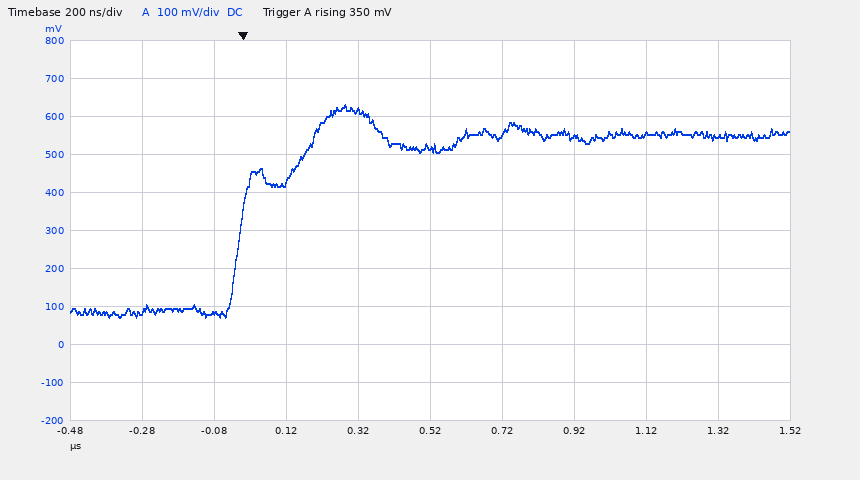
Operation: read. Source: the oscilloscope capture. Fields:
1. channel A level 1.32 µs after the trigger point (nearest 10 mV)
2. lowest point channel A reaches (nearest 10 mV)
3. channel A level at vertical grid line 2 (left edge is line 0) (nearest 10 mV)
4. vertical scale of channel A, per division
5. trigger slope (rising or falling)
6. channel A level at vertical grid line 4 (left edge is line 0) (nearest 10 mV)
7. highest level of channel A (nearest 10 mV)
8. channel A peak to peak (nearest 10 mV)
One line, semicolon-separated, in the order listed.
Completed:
550 mV; 70 mV; 80 mV; 100 mV; rising; 620 mV; 630 mV; 560 mV
